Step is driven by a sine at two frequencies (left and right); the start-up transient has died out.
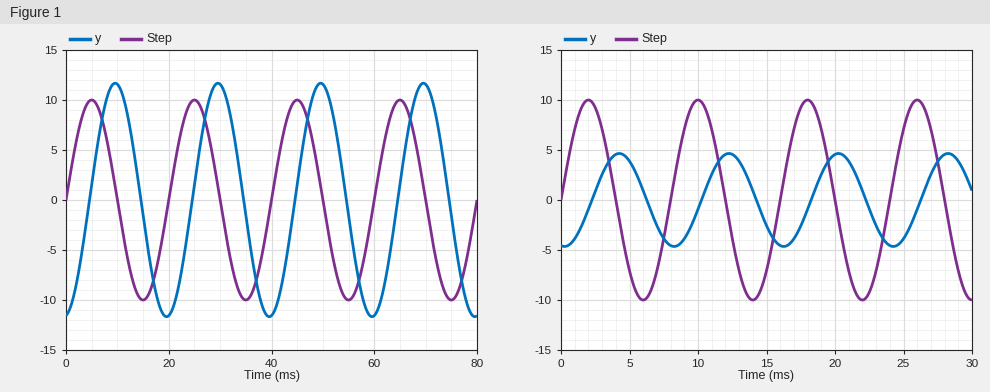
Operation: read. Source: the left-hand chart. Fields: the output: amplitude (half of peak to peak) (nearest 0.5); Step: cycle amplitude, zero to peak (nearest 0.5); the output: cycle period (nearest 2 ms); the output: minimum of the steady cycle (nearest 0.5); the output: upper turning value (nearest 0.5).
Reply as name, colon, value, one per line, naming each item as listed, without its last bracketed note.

the output: amplitude (half of peak to peak): 11.5
Step: cycle amplitude, zero to peak: 10.0
the output: cycle period: 20 ms
the output: minimum of the steady cycle: -11.5
the output: upper turning value: 11.5
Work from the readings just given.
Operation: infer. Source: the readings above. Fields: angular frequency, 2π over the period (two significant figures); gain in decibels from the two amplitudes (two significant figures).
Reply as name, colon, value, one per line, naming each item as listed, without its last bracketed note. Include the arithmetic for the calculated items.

angular frequency, 2π over the period: 2π / 20 = 0.31 rad/ms
gain in decibels from the two amplitudes: 20 log10(11.5 / 10) = 1.2 dB
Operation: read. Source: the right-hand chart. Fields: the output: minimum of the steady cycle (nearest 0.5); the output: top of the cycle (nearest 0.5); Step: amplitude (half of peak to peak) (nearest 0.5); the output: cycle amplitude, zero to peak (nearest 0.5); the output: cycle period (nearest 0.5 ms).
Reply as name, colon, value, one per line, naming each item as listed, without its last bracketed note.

the output: minimum of the steady cycle: -4.5
the output: top of the cycle: 4.5
Step: amplitude (half of peak to peak): 10.0
the output: cycle amplitude, zero to peak: 4.5
the output: cycle period: 8.0 ms
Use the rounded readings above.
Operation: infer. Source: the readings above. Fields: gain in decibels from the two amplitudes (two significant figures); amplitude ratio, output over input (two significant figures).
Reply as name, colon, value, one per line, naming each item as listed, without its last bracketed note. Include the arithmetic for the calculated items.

gain in decibels from the two amplitudes: 20 log10(4.5 / 10) = -6.9 dB
amplitude ratio, output over input: 4.5 / 10 = 0.45
